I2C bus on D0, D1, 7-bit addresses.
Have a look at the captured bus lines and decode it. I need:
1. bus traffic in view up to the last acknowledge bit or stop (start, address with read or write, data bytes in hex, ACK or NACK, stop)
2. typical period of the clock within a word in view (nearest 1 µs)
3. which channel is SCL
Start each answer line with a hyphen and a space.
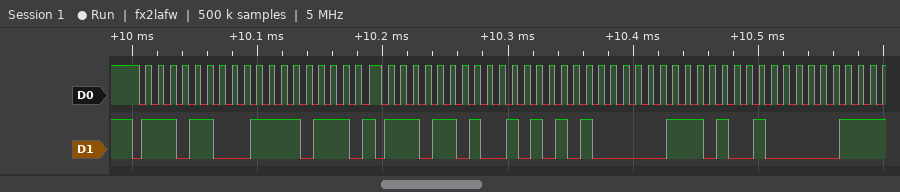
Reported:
- start, address 76 write ACK, F7 ACK, repeated start, address 76 read ACK, 55 ACK, 07 ACK, 90 ACK
- 10 µs
- D0
